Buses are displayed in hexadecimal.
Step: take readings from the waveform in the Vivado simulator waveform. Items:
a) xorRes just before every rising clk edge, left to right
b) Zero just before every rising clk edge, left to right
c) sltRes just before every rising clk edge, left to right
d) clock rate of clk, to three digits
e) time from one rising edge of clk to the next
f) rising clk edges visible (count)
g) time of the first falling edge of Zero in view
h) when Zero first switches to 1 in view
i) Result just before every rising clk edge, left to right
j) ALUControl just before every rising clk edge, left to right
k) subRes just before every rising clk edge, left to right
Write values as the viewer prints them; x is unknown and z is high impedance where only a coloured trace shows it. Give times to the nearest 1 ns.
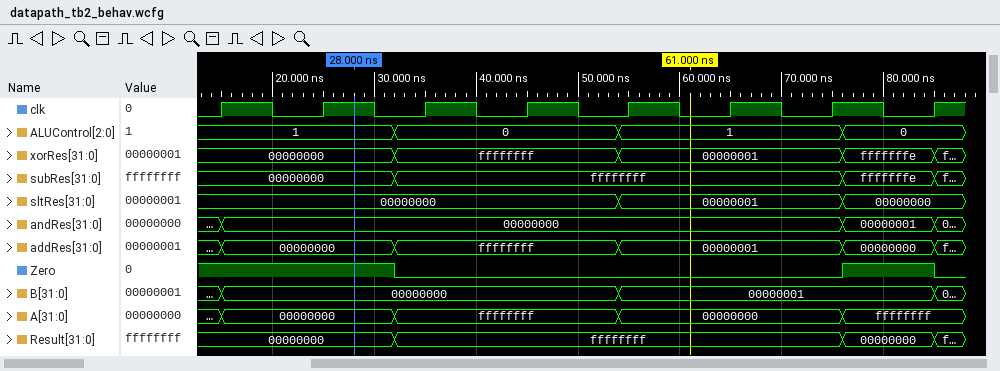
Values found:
00000000, 00000000, ffffffff, ffffffff, 00000001, 00000001, 00000001, fffffffe
1 1 0 0 0 0 0 1
00000000, 00000000, 00000000, 00000000, 00000001, 00000001, 00000001, 00000000
100 MHz
10 ns
8
32 ns
76 ns
00000000, 00000000, ffffffff, ffffffff, ffffffff, ffffffff, ffffffff, 00000000
1, 1, 0, 0, 1, 1, 1, 0
00000000, 00000000, ffffffff, ffffffff, ffffffff, ffffffff, ffffffff, fffffffe
